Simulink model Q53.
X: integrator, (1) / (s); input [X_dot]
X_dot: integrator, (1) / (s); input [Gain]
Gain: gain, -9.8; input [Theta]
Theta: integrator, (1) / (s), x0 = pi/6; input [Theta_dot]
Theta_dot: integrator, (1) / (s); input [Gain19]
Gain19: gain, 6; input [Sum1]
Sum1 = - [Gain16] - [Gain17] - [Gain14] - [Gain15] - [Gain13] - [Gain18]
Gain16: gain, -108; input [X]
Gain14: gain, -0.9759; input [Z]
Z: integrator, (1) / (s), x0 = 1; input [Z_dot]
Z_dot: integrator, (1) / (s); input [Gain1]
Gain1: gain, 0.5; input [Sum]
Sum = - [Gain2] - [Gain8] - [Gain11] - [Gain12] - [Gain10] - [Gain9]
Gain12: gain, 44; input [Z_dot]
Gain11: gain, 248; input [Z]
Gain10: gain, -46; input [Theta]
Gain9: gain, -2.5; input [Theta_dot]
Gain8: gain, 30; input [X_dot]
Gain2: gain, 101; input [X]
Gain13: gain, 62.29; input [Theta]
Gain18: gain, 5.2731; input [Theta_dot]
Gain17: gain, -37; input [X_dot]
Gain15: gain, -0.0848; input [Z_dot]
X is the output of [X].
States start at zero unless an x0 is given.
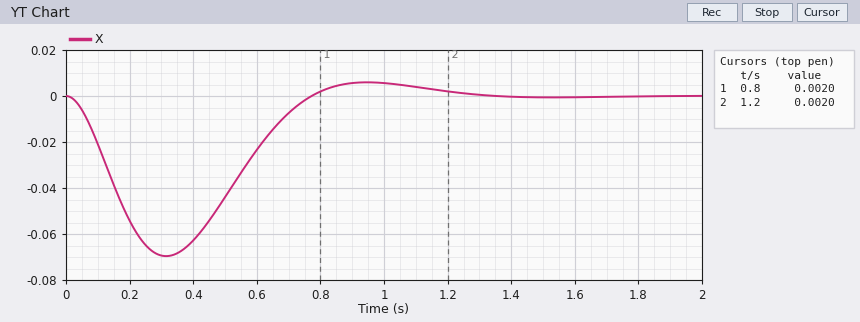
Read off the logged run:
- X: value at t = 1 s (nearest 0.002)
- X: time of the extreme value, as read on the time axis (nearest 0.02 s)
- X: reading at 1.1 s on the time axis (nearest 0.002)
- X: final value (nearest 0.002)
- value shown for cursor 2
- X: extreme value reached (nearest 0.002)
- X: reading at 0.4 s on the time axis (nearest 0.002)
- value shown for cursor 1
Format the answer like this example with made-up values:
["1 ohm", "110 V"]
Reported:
["0.006", "0.32 s", "0.004", "0.000", "0.0020", "-0.070", "-0.062", "0.0020"]
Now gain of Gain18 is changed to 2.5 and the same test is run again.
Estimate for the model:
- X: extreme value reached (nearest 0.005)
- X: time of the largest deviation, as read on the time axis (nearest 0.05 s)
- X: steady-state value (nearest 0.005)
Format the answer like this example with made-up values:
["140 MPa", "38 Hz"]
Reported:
["-0.040", "0.20 s", "0.000"]
